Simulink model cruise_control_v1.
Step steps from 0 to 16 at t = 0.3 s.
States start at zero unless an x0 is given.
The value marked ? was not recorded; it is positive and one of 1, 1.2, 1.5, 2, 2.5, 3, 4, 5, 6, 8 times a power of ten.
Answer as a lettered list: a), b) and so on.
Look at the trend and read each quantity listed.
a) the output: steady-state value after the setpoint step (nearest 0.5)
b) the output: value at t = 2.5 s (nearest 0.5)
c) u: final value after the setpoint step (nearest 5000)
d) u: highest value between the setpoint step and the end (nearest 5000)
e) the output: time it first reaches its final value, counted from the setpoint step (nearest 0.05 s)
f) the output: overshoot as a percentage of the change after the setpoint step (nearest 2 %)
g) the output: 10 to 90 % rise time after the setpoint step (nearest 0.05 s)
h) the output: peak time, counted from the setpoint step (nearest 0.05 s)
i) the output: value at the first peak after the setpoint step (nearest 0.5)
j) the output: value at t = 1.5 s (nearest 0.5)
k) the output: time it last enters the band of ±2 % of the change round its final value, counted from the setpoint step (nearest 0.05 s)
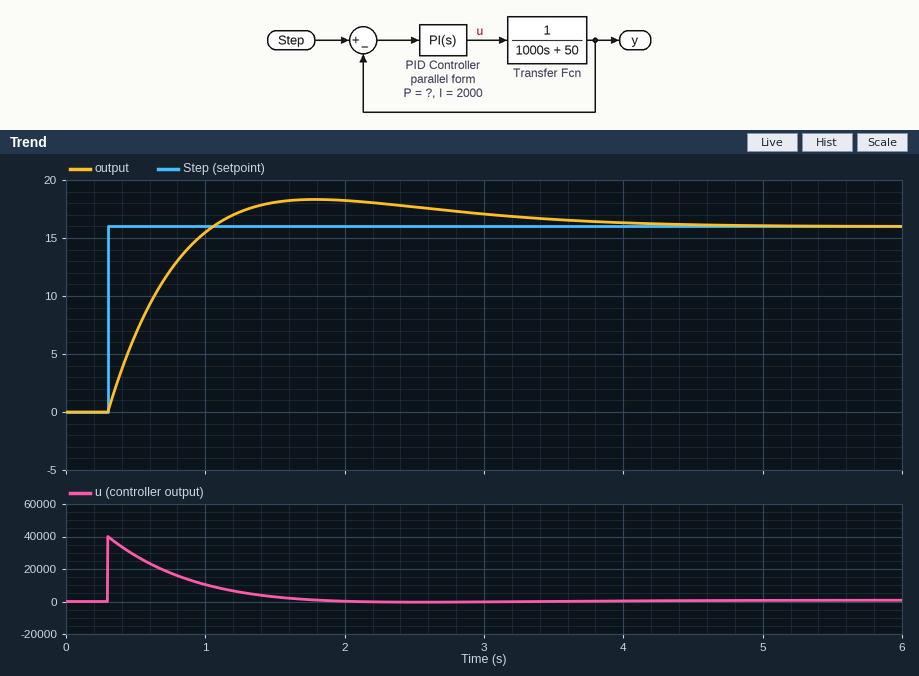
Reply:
a) 16.0
b) 17.5
c) 0
d) 40000
e) 0.75 s
f) 14 %
g) 0.55 s
h) 1.50 s
i) 18.5
j) 18.0
k) 3.70 s
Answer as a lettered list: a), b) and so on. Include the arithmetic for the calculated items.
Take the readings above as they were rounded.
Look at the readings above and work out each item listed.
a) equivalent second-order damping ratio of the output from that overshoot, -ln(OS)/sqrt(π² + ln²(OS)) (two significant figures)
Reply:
a) ln(0.14) = -1.966; 1.966 / sqrt(9.870 + 3.866) = 0.53
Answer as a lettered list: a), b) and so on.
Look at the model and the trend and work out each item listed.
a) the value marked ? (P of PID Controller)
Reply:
a) 2500
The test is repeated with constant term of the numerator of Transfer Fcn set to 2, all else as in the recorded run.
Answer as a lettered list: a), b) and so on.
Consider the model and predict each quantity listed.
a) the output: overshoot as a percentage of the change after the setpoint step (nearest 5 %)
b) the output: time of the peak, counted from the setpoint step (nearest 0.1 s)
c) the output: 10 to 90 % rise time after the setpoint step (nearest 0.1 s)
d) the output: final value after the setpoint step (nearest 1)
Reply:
a) 10 %
b) 0.9 s
c) 0.3 s
d) 16
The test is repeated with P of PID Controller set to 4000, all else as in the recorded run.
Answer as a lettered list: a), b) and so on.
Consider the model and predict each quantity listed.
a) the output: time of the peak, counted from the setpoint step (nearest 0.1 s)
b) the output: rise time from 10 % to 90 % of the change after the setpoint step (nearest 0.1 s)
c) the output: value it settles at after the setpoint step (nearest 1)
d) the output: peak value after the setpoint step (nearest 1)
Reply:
a) 1.3 s
b) 0.4 s
c) 16
d) 17
